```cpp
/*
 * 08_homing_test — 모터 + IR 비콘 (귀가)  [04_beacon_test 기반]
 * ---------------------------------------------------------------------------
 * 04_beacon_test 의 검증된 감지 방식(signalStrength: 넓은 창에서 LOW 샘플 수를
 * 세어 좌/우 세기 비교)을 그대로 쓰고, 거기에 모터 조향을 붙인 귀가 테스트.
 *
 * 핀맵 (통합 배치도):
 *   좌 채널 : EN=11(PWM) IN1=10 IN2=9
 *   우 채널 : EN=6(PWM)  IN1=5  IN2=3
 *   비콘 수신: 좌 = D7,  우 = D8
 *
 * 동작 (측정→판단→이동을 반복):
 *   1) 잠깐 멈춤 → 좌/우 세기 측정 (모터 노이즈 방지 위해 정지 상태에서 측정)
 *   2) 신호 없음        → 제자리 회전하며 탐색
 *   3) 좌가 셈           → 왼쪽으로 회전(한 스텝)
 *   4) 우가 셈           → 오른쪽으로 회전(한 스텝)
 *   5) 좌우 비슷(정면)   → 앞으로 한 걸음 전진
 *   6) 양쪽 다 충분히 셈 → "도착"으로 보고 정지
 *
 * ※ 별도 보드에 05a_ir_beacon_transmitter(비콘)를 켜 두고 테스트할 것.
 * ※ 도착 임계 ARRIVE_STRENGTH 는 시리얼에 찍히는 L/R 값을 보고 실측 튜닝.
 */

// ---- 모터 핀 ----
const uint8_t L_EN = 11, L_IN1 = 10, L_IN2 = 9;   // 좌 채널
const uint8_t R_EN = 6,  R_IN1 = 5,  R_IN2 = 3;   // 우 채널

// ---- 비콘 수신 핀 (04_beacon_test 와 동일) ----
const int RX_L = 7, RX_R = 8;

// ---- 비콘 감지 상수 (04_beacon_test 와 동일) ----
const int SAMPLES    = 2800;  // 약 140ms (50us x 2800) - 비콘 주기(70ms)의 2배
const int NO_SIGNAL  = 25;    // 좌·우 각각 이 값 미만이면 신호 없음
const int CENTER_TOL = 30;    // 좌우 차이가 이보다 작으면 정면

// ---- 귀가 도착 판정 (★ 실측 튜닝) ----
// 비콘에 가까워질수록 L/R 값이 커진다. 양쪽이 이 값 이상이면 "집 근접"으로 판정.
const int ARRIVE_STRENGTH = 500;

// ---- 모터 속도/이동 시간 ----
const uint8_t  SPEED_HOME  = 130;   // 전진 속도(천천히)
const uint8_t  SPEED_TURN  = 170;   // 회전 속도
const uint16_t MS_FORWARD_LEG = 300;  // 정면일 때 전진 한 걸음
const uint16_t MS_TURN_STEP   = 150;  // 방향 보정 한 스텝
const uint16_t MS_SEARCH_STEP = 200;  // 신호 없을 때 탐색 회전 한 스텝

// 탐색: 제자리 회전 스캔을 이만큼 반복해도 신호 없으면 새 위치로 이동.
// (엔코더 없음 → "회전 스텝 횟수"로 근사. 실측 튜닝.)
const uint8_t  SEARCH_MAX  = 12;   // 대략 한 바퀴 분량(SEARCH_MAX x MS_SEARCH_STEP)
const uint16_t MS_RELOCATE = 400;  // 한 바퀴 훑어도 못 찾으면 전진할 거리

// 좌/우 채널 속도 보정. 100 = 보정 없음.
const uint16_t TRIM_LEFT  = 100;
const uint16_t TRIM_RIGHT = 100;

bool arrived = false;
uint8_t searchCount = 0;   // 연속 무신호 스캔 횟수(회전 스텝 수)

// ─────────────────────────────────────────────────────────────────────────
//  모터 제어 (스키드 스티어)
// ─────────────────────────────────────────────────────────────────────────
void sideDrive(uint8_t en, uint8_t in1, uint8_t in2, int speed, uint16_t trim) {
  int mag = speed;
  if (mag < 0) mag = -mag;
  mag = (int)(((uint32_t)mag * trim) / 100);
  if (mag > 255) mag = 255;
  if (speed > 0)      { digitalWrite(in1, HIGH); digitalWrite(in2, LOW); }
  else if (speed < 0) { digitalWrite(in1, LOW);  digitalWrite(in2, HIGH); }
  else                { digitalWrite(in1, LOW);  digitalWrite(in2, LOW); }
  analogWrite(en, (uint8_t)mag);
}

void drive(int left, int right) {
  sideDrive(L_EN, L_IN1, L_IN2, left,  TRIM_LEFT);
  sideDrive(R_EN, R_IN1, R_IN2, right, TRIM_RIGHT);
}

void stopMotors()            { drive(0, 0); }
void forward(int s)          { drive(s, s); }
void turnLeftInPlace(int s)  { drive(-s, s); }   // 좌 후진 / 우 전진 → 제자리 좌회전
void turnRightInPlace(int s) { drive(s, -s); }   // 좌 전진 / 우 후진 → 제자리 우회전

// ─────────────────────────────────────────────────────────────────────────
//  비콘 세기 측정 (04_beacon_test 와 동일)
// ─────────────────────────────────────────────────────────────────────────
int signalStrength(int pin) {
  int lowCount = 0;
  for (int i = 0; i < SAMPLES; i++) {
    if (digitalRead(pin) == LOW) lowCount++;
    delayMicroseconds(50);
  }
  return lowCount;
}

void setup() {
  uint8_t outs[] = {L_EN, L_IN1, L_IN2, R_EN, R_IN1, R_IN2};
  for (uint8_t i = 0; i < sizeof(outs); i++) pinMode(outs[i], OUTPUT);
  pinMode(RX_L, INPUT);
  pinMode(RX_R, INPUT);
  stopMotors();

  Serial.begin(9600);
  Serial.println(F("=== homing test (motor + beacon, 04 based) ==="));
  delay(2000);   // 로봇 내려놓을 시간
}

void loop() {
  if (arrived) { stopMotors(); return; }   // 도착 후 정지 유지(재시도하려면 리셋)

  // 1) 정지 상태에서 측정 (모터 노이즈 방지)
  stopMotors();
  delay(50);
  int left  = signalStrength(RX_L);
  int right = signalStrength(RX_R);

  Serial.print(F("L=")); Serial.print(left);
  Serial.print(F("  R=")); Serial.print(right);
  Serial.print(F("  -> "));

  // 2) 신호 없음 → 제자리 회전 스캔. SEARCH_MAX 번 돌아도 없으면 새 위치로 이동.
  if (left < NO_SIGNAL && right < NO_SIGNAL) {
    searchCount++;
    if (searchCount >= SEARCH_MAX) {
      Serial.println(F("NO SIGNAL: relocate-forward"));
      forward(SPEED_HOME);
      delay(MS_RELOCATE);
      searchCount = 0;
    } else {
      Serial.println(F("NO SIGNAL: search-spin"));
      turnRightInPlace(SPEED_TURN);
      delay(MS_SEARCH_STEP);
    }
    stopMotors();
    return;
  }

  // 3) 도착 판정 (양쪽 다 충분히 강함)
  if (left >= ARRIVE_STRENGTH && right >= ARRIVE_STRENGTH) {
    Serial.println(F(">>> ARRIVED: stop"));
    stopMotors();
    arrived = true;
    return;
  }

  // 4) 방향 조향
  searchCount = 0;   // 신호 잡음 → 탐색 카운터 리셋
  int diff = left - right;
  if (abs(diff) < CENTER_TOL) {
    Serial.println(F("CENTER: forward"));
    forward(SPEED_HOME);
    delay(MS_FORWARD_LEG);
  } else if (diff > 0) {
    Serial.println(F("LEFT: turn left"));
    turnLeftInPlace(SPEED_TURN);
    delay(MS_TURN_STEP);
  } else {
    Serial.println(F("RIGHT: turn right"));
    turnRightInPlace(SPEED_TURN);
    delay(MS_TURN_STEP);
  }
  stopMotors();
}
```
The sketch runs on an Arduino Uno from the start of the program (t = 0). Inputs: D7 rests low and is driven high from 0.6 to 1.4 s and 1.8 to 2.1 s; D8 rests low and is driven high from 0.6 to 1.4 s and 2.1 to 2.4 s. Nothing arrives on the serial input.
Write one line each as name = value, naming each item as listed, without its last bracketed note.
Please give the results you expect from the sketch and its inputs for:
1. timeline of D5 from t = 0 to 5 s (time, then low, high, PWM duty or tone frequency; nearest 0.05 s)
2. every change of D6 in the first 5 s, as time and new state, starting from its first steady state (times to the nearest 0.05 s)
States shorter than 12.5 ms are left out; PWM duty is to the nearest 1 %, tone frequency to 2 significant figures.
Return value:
timeline of D5 from t = 0 to 5 s = 0 s low; 2.35 s high; 2.5 s low
every change of D6 in the first 5 s, as time and new state, starting from its first steady state = 0 s low; 2.35 s PWM 67 %; 2.5 s low
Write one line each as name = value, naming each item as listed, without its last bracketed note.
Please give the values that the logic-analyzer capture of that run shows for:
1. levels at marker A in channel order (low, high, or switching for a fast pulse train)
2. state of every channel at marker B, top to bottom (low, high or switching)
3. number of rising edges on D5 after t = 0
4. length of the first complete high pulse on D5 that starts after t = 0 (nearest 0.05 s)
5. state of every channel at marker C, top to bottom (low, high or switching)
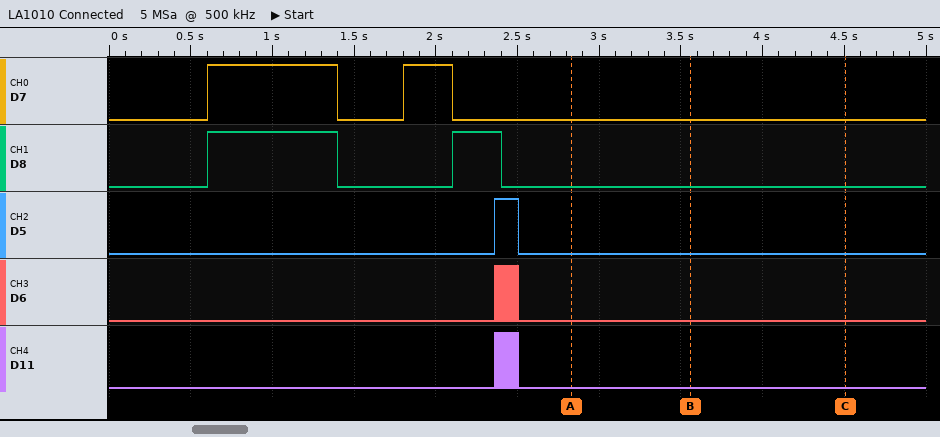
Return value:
levels at marker A in channel order = D7 low, D8 low, D5 low, D6 low, D11 low
state of every channel at marker B, top to bottom = D7 low, D8 low, D5 low, D6 low, D11 low
number of rising edges on D5 after t = 0 = 1
length of the first complete high pulse on D5 that starts after t = 0 = 0.15 s
state of every channel at marker C, top to bottom = D7 low, D8 low, D5 low, D6 low, D11 low
